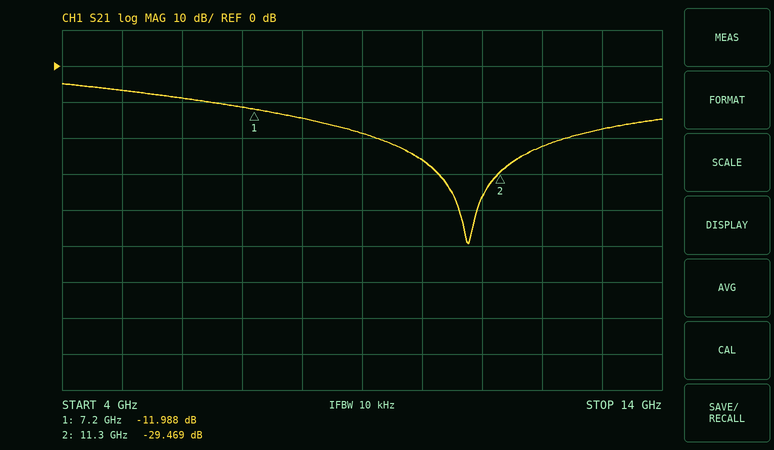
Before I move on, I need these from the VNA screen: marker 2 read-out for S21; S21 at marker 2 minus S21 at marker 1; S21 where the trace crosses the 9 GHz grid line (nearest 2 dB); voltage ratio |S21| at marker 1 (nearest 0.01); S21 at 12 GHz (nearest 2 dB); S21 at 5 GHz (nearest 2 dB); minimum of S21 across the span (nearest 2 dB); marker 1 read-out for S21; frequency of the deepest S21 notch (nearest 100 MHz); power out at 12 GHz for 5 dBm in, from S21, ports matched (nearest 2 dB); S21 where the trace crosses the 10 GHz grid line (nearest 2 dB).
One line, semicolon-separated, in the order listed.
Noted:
-29.469 dB; -17.481 dB; -18 dB; 0.25; -22 dB; -6 dB; -50 dB; -11.988 dB; 10.8 GHz; -18 dBm; -26 dB
